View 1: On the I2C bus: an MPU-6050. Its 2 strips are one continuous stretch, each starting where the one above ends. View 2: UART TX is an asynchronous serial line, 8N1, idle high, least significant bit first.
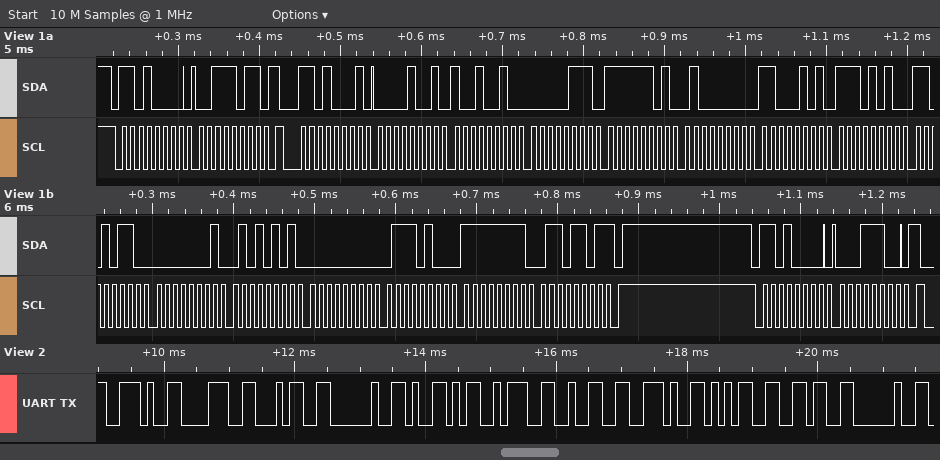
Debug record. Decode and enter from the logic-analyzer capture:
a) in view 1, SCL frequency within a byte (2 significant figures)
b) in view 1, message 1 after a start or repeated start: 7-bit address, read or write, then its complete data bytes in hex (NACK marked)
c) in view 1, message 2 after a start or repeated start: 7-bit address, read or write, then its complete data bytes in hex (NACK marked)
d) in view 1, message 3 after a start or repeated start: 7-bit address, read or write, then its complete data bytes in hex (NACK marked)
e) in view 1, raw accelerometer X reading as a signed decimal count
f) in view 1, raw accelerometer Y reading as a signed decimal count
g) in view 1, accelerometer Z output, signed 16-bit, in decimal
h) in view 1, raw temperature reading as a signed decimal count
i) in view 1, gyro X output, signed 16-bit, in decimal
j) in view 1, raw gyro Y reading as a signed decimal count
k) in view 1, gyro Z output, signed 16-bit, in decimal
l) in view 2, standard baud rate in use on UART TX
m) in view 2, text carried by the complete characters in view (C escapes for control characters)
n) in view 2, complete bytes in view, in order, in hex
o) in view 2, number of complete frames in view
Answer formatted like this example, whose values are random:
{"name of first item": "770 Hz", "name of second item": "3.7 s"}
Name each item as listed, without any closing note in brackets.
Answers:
{"in view 1, SCL frequency within a byte": "100 kHz", "in view 1, message 1 after a start or repeated start: 7-bit address, read or write, then its complete data bytes in hex": "0x68 write: 3B", "in view 1, message 2 after a start or repeated start: 7-bit address, read or write, then its complete data bytes in hex": "0x68 read: 09 92 07 FD 40 C5 EA D6 01 55 00 74 FF 6D NACK", "in view 1, message 3 after a start or repeated start: 7-bit address, read or write, then its complete data bytes in hex": "0x68 write: 1C", "in view 1, raw accelerometer X reading as a signed decimal count": "2450", "in view 1, raw accelerometer Y reading as a signed decimal count": "2045", "in view 1, accelerometer Z output, signed 16-bit, in decimal": "16581", "in view 1, raw temperature reading as a signed decimal count": "-5418", "in view 1, gyro X output, signed 16-bit, in decimal": "341", "in view 1, raw gyro Y reading as a signed decimal count": "116", "in view 1, gyro Z output, signed 16-bit, in decimal": "-147", "in view 2, standard baud rate in use on UART TX": "9600 baud", "in view 2, text carried by the complete characters in view": "\".84 Y:2.56 \"", "in view 2, complete bytes in view, in order, in hex": "2E 38 34 20 59 3A 32 2E 35 36 20", "in view 2, number of complete frames in view": "11"}
